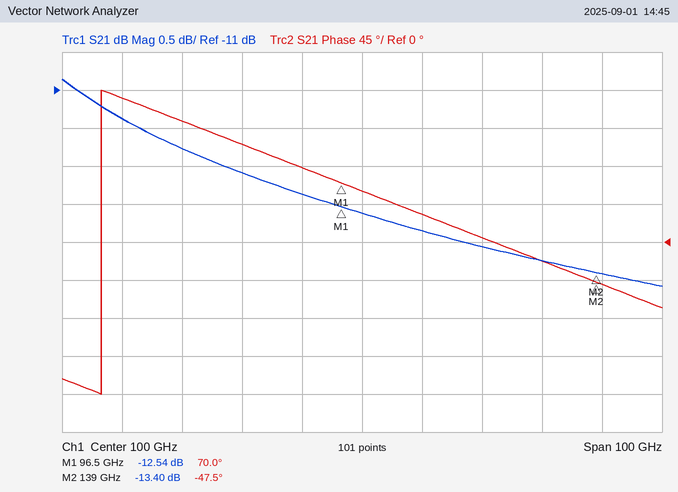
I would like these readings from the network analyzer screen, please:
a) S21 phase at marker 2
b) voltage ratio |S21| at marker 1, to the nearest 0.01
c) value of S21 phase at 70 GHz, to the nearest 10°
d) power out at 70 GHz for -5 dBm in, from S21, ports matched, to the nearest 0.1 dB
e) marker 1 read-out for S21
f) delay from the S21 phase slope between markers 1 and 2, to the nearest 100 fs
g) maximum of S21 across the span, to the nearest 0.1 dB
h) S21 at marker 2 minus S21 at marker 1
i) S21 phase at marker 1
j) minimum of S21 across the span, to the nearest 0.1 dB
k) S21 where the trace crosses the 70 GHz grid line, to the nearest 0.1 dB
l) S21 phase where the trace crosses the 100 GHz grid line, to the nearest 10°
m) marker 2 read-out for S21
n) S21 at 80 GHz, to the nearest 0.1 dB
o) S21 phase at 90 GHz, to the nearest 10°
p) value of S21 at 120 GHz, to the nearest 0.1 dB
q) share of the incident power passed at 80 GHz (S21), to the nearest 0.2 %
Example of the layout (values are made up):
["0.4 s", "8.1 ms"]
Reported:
["-47.5°", "0.24", "140°", "-16.8 dBm", "-12.54 dB", "7.7 ps", "-10.9 dB", "-0.86 dB", "70.0°", "-13.6 dB", "-11.8 dB", "60°", "-13.40 dB", "-12.1 dB", "90°", "-13.1 dB", "6.2 %"]
